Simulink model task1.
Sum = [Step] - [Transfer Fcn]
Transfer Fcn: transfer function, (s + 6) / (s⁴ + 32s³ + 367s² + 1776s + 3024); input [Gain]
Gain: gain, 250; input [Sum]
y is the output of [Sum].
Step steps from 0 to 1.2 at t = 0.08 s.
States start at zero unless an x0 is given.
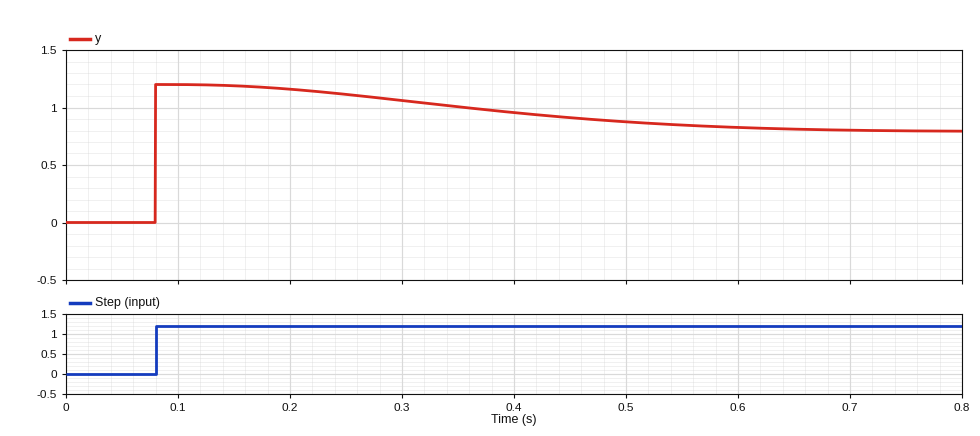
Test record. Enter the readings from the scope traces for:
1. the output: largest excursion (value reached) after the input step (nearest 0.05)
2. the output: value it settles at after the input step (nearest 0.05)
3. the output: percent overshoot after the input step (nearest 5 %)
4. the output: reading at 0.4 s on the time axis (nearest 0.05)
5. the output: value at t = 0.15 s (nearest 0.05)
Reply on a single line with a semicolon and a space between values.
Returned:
1.20; 0.80; 50 %; 0.95; 1.20
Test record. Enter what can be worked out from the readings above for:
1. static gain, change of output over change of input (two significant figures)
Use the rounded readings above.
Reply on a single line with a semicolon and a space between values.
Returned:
0.67
